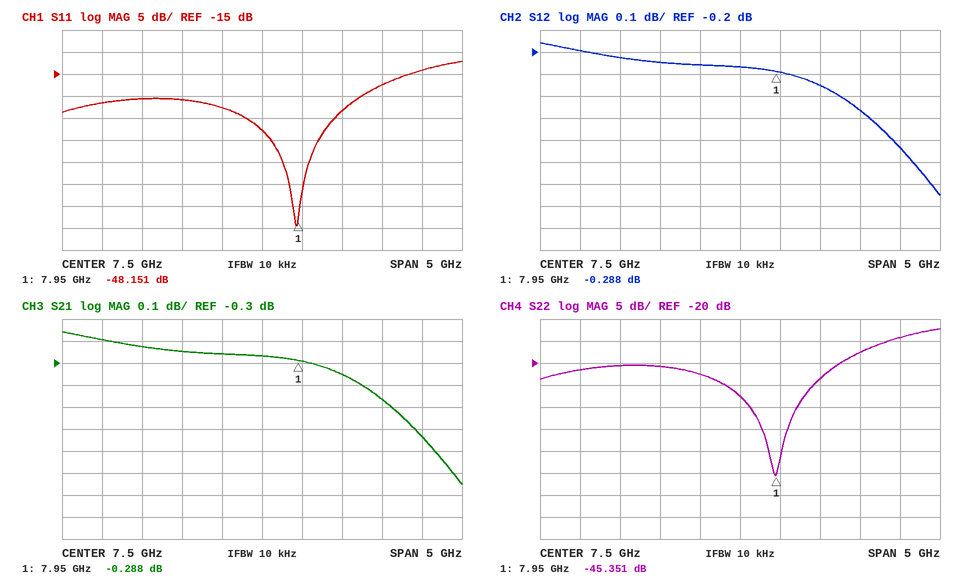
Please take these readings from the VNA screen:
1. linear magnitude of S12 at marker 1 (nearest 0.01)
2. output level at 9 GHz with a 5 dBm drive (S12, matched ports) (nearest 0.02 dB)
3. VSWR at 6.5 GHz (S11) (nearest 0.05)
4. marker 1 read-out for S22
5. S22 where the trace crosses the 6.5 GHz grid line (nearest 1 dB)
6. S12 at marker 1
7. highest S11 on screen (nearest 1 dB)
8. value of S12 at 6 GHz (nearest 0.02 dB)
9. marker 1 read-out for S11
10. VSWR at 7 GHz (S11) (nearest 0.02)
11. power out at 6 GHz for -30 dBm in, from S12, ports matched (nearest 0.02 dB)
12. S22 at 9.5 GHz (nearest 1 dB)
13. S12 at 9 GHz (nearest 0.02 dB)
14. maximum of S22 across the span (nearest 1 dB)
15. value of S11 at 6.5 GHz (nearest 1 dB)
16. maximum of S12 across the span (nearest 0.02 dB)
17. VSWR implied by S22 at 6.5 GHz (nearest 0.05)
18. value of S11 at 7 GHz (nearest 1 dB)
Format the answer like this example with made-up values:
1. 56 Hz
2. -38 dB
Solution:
1. 0.97
2. 4.54 dBm
3. 1.20
4. -45.351 dB
5. -21 dB
6. -0.288 dB
7. -12 dB
8. -0.22 dB
9. -48.151 dB
10. 1.16
11. -30.22 dBm
12. -14 dB
13. -0.46 dB
14. -12 dB
15. -21 dB
16. -0.16 dB
17. 1.20
18. -23 dB
